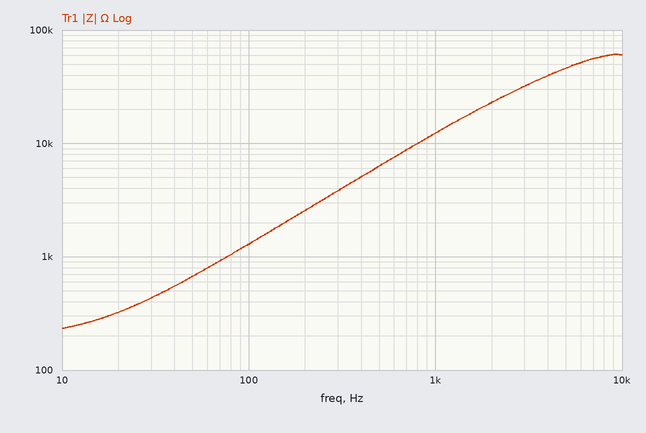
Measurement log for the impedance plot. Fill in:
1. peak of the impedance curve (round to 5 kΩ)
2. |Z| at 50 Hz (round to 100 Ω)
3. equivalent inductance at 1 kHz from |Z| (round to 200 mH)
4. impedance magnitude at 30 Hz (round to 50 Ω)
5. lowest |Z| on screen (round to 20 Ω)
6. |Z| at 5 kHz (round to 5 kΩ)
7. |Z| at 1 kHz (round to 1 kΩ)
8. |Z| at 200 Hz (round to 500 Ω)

60 kΩ
700 Ω
2.0 H
450 Ω
240 Ω
45 kΩ
12 kΩ
2.5 kΩ
